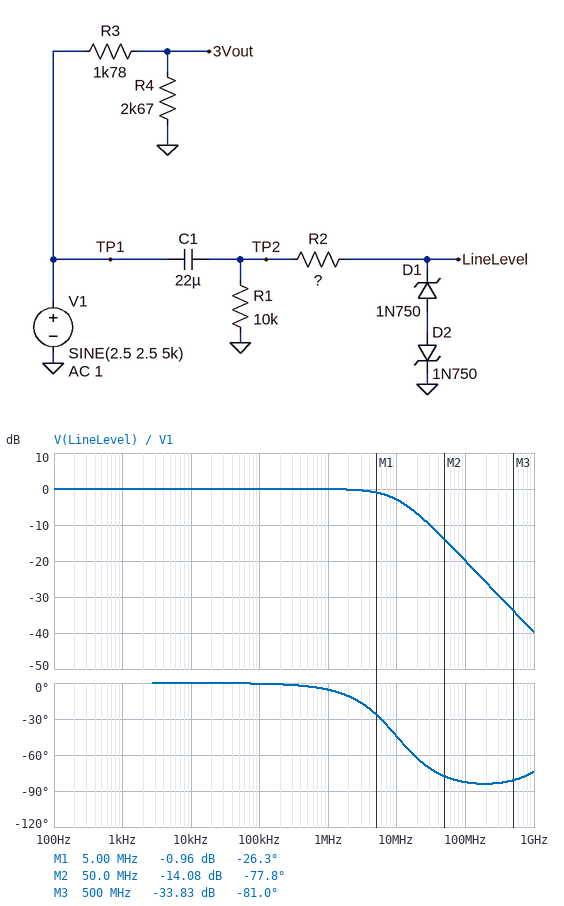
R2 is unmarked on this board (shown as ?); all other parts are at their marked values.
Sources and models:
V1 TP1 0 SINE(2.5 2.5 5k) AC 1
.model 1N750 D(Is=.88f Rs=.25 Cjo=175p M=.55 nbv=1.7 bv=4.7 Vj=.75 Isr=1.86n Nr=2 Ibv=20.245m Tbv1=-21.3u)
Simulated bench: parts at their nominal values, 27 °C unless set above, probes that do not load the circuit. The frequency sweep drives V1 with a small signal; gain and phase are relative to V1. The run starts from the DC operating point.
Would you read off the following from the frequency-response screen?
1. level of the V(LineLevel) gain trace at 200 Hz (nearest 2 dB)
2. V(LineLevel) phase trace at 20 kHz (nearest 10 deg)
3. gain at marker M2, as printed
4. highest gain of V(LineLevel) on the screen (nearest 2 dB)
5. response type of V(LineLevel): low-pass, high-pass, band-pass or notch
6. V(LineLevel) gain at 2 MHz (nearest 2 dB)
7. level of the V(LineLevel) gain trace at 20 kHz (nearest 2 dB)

0 dB
0 deg
-14.08 dB
0 dB
low-pass
0 dB
0 dB
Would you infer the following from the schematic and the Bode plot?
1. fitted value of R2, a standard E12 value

180 Ω
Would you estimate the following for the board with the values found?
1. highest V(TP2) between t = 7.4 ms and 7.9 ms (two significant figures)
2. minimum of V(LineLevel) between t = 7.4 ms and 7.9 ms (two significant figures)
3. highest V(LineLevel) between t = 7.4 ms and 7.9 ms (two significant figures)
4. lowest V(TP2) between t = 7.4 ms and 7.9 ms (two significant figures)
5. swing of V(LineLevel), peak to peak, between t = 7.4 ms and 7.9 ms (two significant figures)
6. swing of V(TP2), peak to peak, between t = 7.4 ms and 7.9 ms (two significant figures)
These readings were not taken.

2.5 V
-2.5 V
2.5 V
-2.5 V
5.0 V
5.0 V
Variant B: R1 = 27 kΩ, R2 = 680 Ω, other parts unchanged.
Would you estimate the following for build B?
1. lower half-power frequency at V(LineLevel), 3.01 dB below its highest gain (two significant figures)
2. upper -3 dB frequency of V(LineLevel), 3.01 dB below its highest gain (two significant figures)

270 mHz
2.7 MHz
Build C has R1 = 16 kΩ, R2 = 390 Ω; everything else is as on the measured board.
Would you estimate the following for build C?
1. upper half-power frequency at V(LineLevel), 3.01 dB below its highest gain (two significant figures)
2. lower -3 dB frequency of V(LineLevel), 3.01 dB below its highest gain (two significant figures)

4.7 MHz
450 mHz
